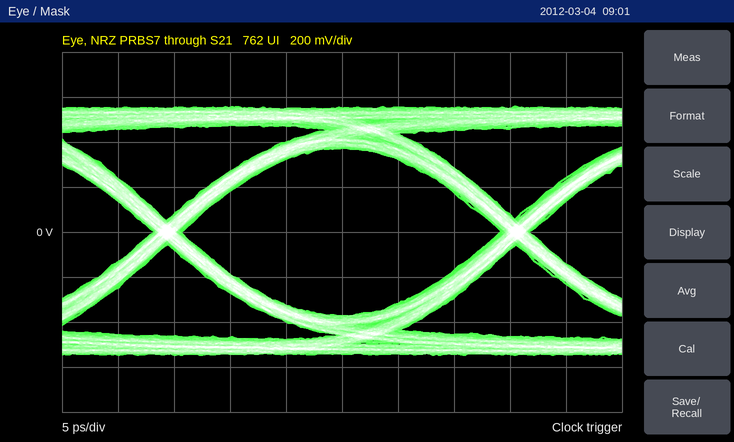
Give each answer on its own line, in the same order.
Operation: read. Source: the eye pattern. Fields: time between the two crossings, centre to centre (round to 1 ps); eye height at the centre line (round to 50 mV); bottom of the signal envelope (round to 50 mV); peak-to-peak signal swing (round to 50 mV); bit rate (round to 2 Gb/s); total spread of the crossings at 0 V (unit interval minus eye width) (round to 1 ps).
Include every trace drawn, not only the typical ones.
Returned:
31 ps
750 mV
-550 mV
1.10 V
32 Gb/s
3 ps
